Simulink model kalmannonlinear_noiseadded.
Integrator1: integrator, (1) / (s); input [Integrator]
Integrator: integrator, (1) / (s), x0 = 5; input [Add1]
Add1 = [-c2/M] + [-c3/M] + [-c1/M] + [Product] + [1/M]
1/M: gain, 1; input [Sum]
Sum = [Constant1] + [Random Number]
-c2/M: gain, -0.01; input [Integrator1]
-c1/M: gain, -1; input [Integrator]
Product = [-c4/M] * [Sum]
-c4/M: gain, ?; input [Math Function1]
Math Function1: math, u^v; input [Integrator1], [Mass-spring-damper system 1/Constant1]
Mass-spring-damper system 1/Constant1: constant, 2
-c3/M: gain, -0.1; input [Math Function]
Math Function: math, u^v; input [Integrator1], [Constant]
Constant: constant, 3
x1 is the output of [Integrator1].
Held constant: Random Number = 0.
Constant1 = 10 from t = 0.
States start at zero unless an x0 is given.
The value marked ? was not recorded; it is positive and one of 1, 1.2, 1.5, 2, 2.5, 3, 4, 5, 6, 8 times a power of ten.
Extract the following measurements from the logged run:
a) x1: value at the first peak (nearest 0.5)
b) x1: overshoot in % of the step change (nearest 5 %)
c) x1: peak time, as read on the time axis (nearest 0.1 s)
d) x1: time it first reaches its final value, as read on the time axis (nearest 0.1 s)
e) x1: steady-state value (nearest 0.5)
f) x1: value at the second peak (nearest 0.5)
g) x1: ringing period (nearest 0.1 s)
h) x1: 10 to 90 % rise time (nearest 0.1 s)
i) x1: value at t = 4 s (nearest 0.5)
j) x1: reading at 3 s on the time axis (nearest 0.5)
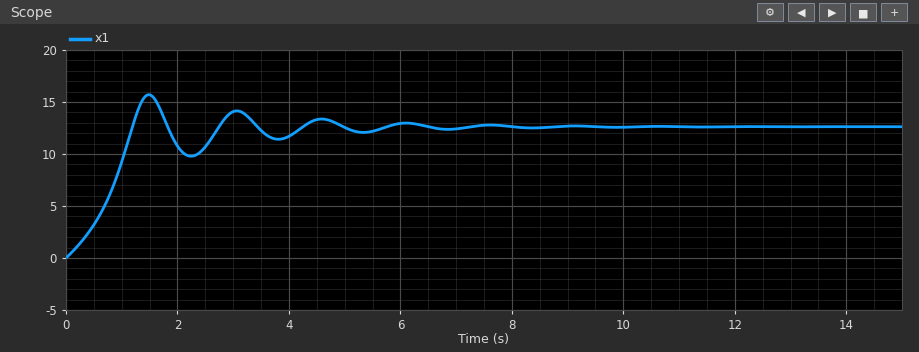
15.5
25 %
1.5 s
1.2 s
12.5
14.0
1.6 s
0.9 s
11.5
14.0
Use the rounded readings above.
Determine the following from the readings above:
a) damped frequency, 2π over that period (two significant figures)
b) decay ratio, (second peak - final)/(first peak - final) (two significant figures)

3.9 rad/s
0.50
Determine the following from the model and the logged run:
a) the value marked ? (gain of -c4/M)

0.12
